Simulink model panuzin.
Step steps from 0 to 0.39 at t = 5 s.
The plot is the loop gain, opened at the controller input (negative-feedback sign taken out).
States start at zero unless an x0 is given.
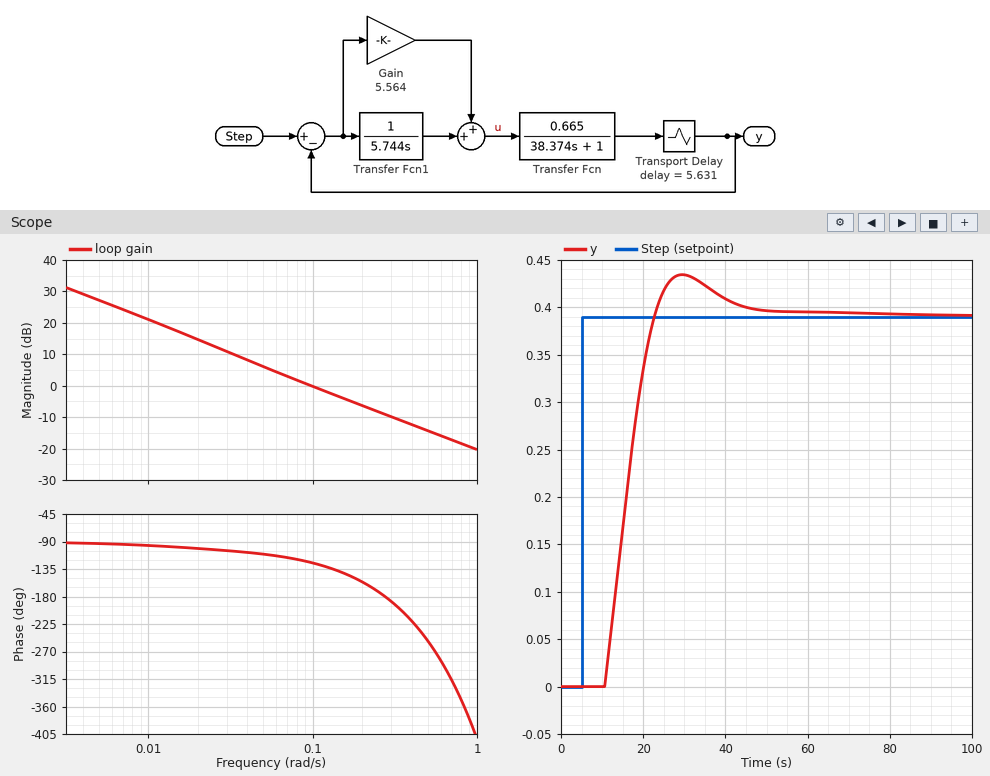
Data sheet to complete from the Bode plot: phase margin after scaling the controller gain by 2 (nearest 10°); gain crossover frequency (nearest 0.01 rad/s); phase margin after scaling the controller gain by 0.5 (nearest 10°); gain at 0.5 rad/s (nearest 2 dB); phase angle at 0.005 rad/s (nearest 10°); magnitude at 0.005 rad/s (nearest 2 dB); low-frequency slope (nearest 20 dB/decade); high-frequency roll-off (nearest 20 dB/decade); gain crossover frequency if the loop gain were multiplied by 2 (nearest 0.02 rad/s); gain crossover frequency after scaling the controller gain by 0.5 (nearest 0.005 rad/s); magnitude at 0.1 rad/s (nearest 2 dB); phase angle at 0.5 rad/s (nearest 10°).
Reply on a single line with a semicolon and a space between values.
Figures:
30°; 0.10 rad/s; 70°; -14 dB; -90°; 28 dB; -20 dB/decade; -20 dB/decade; 0.20 rad/s; 0.050 rad/s; 0 dB; -250°
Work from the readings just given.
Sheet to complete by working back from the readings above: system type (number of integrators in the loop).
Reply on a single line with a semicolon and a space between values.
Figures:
1
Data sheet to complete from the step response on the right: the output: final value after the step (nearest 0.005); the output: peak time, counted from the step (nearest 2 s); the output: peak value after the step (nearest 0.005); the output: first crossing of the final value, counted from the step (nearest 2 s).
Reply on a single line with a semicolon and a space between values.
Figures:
0.390; 24 s; 0.435; 18 s
